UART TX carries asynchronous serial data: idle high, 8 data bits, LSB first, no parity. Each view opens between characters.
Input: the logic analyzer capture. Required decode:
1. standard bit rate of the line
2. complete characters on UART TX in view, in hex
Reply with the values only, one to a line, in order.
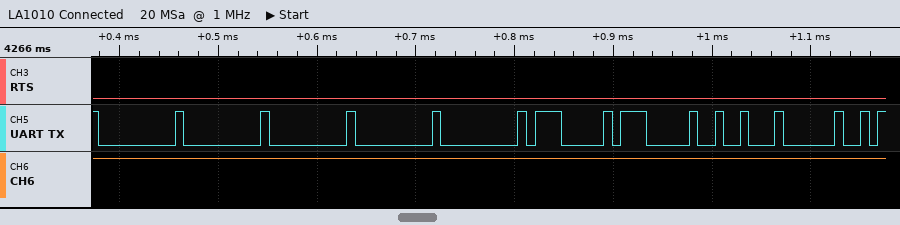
115200 baud
00, 00, 00, 00, 00, 07, 07, 12, 20
